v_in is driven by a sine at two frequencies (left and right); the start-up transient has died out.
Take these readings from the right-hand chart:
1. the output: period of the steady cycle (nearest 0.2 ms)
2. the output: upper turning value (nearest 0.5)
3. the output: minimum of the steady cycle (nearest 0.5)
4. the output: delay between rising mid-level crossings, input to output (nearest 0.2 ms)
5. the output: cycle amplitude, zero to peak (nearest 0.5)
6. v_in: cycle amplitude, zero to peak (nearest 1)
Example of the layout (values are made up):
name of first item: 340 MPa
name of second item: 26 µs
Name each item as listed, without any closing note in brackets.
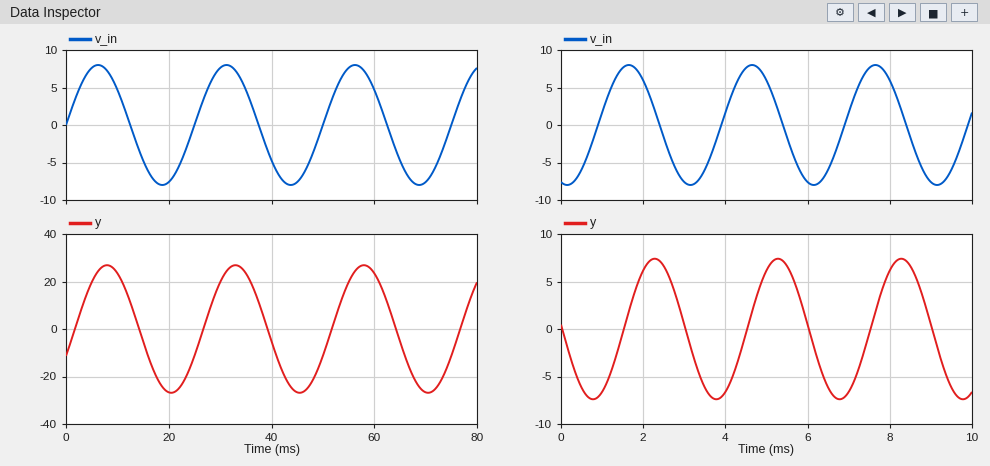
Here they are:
the output: period of the steady cycle: 3.0 ms
the output: upper turning value: 7.5
the output: minimum of the steady cycle: -7.5
the output: delay between rising mid-level crossings, input to output: 0.6 ms
the output: cycle amplitude, zero to peak: 7.5
v_in: cycle amplitude, zero to peak: 8
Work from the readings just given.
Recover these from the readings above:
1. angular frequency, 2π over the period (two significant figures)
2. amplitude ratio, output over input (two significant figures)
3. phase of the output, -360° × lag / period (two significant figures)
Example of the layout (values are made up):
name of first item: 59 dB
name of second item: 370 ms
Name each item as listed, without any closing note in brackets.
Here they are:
angular frequency, 2π over the period: 2.1 rad/ms
amplitude ratio, output over input: 0.94
phase of the output, -360° × lag / period: -72°
